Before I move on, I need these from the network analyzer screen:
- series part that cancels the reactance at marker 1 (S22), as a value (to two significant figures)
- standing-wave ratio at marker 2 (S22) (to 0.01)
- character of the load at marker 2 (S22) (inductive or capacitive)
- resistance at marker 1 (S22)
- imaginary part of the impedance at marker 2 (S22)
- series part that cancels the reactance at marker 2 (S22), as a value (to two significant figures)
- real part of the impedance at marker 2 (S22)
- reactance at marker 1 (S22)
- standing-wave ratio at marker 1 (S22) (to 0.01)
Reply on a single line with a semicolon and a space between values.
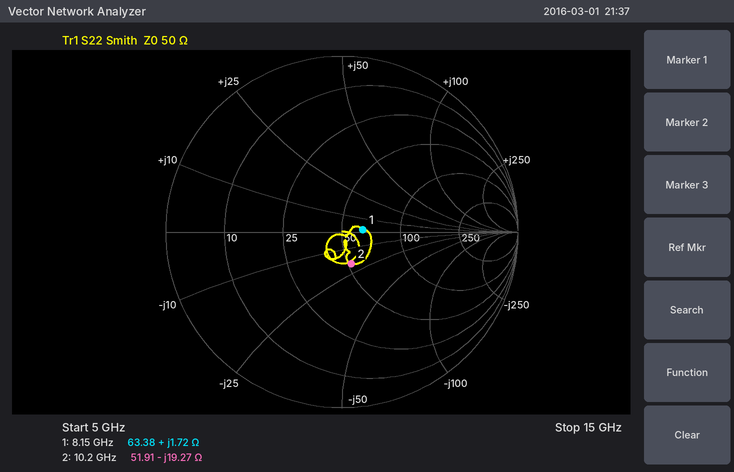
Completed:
11 pF; 1.46; capacitive; 63.38 Ω; -19.27 Ω; 300 pH; 51.91 Ω; +1.72 Ω; 1.27
